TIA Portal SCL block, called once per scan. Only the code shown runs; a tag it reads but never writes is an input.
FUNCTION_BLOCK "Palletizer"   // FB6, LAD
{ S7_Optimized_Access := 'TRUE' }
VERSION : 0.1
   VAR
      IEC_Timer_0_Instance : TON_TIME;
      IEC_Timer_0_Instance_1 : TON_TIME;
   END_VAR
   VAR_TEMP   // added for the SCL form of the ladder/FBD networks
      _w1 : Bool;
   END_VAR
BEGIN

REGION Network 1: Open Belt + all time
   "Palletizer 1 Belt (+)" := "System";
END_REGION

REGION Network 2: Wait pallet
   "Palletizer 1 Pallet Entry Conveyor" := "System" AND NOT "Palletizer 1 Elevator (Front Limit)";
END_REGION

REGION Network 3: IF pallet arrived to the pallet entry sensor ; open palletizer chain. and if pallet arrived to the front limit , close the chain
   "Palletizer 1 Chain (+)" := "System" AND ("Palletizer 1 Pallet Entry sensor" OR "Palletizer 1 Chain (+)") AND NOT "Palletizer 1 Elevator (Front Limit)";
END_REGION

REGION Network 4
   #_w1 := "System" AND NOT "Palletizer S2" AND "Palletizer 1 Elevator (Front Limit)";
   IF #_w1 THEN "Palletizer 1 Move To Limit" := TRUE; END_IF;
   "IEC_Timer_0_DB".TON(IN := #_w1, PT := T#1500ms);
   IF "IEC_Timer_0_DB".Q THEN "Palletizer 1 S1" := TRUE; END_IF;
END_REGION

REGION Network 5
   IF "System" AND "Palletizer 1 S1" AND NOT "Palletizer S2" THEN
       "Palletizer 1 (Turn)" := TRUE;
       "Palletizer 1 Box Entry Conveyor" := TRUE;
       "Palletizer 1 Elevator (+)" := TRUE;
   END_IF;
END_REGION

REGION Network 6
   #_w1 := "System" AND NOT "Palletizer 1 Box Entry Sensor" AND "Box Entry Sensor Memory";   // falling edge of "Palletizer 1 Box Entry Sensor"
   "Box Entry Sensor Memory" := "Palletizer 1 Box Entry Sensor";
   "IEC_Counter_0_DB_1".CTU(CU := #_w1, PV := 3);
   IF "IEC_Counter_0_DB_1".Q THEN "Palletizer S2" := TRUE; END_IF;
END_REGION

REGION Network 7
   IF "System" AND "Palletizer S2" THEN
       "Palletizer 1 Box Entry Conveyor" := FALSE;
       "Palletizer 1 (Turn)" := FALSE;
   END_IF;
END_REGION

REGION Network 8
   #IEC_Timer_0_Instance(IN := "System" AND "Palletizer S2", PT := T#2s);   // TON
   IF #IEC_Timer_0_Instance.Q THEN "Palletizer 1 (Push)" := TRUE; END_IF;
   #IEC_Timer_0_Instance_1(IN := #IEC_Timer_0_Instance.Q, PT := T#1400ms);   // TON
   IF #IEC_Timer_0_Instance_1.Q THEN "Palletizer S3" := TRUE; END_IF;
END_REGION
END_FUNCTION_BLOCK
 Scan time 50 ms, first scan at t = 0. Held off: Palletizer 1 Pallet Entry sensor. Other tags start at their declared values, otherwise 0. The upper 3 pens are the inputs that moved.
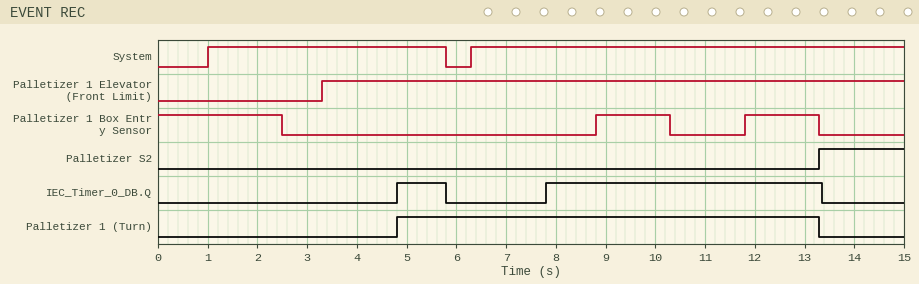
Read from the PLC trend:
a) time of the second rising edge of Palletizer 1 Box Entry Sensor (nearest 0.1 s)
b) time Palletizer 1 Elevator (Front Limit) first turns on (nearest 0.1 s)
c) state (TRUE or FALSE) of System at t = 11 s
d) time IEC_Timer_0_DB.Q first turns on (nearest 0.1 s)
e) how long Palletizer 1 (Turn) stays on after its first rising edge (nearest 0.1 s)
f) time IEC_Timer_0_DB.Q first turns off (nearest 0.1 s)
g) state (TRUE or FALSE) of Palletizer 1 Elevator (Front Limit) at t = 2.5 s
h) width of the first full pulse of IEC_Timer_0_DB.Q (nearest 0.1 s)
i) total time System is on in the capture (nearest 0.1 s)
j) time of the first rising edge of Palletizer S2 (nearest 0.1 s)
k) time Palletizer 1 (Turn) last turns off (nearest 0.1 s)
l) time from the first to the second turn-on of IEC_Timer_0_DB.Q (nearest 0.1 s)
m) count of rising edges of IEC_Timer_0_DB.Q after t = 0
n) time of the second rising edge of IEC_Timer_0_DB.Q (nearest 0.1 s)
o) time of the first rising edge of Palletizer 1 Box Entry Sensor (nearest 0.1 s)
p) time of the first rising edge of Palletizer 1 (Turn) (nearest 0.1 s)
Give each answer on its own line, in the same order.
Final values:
11.8 s
3.3 s
TRUE
4.8 s
8.5 s
5.8 s
FALSE
1.0 s
13.5 s
13.3 s
13.3 s
3.0 s
2
7.8 s
8.8 s
4.8 s
